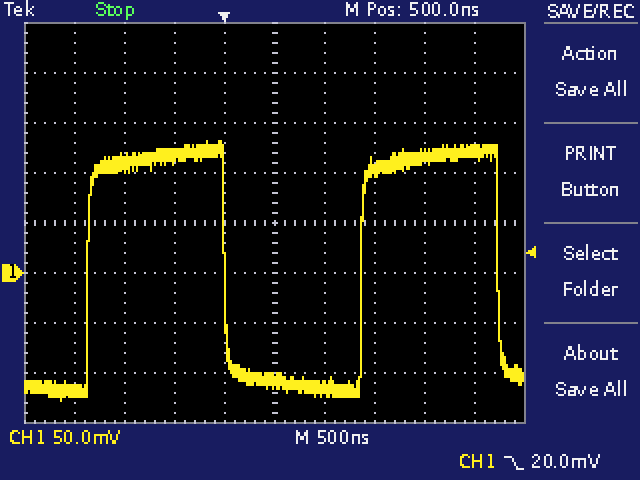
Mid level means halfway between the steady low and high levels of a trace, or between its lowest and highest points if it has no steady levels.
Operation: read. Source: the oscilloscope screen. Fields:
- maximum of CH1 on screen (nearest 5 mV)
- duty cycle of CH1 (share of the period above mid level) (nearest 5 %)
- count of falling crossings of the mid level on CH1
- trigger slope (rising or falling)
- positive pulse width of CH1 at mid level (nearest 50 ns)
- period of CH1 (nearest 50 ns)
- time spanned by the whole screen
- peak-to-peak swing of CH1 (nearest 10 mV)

130 mV
50 %
2
falling
1.35 µs
2.75 µs
5 µs
260 mV
